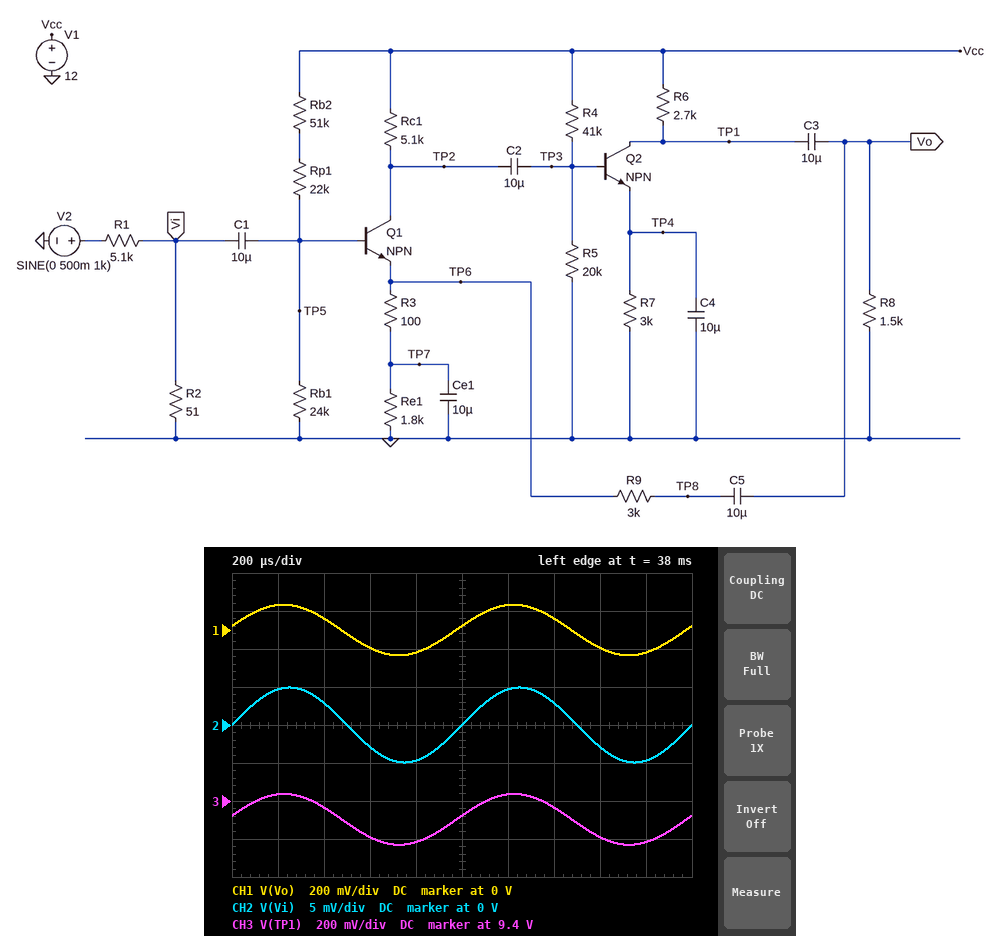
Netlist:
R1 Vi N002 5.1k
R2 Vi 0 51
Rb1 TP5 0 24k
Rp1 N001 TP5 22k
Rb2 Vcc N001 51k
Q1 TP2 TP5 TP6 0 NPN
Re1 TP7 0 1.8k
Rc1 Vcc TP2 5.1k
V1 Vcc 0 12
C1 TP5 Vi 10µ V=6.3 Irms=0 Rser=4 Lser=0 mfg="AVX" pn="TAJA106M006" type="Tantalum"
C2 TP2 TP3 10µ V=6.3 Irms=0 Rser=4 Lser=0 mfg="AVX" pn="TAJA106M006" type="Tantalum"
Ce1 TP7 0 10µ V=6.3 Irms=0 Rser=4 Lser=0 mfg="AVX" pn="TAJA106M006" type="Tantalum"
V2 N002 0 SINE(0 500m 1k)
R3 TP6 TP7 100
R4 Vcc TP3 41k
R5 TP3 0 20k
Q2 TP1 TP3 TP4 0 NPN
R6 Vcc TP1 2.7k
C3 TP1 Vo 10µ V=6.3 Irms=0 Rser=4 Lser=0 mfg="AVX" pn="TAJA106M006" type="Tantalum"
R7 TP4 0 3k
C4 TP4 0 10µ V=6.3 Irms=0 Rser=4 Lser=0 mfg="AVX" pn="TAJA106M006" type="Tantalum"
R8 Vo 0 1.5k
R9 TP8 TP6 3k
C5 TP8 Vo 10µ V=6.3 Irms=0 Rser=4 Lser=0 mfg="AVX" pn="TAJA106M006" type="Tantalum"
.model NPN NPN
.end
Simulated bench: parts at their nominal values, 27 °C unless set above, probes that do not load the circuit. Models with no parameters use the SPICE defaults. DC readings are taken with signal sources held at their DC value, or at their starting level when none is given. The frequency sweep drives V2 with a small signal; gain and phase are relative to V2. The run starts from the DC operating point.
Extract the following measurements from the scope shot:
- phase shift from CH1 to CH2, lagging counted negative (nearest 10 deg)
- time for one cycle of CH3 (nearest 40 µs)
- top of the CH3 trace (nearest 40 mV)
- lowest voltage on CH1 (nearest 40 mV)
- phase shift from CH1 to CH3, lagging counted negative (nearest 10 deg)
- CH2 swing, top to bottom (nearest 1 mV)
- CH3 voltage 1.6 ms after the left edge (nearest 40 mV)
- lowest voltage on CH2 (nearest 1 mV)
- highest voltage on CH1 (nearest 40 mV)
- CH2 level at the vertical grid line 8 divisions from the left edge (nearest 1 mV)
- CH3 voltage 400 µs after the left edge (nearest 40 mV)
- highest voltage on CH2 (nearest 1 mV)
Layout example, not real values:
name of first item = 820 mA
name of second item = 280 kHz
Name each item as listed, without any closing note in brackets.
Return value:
phase shift from CH1 to CH2, lagging counted negative = -10 deg
time for one cycle of CH3 = 1.00 ms
top of the CH3 trace = 9.44 V
lowest voltage on CH1 = -120 mV
phase shift from CH1 to CH3, lagging counted negative = 0 deg
CH2 swing, top to bottom = 10 mV
CH3 voltage 1.6 ms after the left edge = 9.20 V
lowest voltage on CH2 = -5 mV
highest voltage on CH1 = 120 mV
CH2 level at the vertical grid line 8 divisions from the left edge = -3 mV
CH3 voltage 400 µs after the left edge = 9.36 V
highest voltage on CH2 = 5 mV
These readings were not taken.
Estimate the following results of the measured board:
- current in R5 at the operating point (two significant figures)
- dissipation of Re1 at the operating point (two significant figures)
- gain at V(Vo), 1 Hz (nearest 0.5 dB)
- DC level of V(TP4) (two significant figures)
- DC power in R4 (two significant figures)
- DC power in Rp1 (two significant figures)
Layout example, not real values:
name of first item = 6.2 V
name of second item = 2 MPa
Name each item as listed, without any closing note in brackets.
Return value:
current in R5 at the operating point = 190 µA
dissipation of Re1 at the operating point = 2.0 mW
gain at V(Vo), 1 Hz = -58.0 dB
DC level of V(TP4) = 3.0 V
DC power in R4 = 1.6 mW
DC power in Rp1 = 350 µW
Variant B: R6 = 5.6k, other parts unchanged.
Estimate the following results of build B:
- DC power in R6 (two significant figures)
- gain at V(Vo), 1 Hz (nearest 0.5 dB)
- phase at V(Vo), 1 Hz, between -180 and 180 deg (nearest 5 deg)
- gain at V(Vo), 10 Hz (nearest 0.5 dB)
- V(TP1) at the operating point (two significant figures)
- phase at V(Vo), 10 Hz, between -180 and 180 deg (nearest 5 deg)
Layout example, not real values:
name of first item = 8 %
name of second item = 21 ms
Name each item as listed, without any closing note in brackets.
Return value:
DC power in R6 = 5.6 mW
gain at V(Vo), 1 Hz = -53.5 dB
phase at V(Vo), 1 Hz, between -180 and 180 deg = 155 deg
gain at V(Vo), 10 Hz = -34.0 dB
V(TP1) at the operating point = 6.4 V
phase at V(Vo), 10 Hz, between -180 and 180 deg = 75 deg
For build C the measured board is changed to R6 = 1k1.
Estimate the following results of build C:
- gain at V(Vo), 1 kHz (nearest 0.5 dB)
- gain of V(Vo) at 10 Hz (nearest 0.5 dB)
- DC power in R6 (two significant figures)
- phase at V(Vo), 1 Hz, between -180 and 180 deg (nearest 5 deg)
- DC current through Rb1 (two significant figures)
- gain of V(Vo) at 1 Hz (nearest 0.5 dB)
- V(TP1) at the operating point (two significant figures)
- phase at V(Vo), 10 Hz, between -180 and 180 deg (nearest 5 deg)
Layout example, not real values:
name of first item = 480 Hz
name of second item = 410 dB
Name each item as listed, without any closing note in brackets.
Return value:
gain at V(Vo), 1 kHz = -12.0 dB
gain of V(Vo) at 10 Hz = -39.0 dB
DC power in R6 = 1.1 mW
phase at V(Vo), 1 Hz, between -180 and 180 deg = 135 deg
DC current through Rb1 = 120 µA
gain of V(Vo) at 1 Hz = -62.0 dB
V(TP1) at the operating point = 11 V
phase at V(Vo), 10 Hz, between -180 and 180 deg = 115 deg
